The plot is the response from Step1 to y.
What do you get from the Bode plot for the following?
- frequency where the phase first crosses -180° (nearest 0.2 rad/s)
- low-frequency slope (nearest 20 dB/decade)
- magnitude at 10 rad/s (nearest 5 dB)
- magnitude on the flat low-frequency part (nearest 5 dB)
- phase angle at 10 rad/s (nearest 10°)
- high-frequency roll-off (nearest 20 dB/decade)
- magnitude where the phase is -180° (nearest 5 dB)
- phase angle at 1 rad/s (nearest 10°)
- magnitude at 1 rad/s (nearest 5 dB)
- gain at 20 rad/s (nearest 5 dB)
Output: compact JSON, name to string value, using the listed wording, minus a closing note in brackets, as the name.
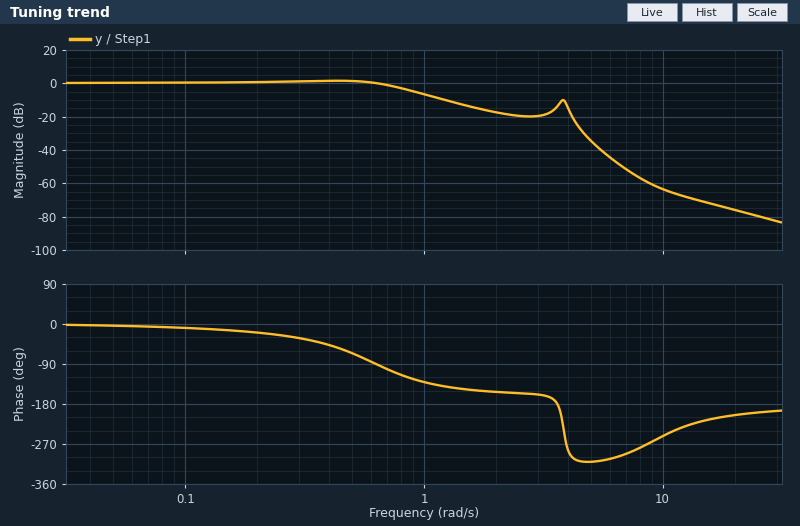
{"frequency where the phase first crosses -180°": "3.6 rad/s", "low-frequency slope": "0 dB/decade", "magnitude at 10 rad/s": "-65 dB", "magnitude on the flat low-frequency part": "0 dB", "phase angle at 10 rad/s": "-250°", "high-frequency roll-off": "-40 dB/decade", "magnitude where the phase is -180°": "-15 dB", "phase angle at 1 rad/s": "-130°", "magnitude at 1 rad/s": "-5 dB", "gain at 20 rad/s": "-75 dB"}
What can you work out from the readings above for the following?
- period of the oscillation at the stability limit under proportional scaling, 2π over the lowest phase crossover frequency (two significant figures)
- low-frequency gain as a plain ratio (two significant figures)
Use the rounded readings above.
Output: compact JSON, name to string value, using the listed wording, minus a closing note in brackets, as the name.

{"period of the oscillation at the stability limit under proportional scaling, 2π over the lowest phase crossover frequency": "1.7 s", "low-frequency gain as a plain ratio": "1.0"}
